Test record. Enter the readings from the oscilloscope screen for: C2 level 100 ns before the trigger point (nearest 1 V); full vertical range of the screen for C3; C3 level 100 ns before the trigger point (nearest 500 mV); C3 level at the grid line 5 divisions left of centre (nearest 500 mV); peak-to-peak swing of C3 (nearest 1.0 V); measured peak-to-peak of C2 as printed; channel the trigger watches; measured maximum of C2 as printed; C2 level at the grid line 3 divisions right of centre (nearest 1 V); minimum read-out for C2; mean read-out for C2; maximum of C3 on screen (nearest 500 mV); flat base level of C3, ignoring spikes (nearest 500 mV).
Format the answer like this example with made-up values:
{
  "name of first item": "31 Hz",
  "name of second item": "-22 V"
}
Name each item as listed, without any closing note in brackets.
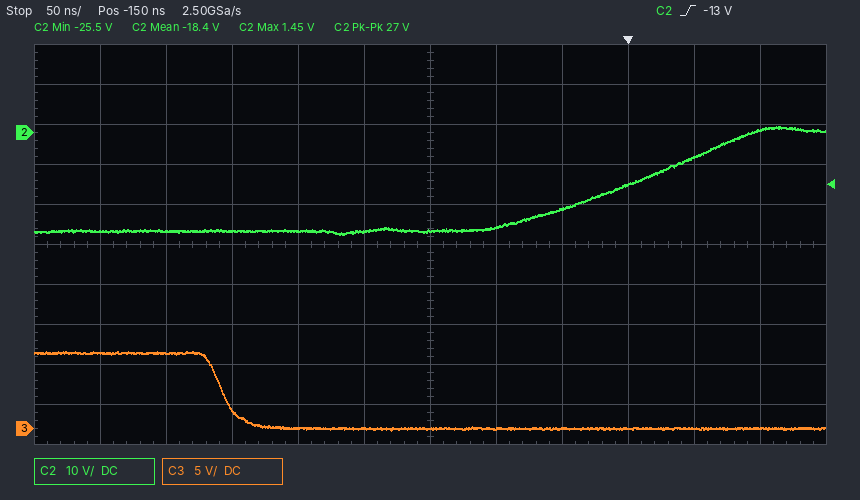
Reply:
{
  "C2 level 100 ns before the trigger point": "-24 V",
  "full vertical range of the screen for C3": "50 V",
  "C3 level 100 ns before the trigger point": "0.0 V",
  "C3 level at the grid line 5 divisions left of centre": "9.5 V",
  "peak-to-peak swing of C3": "10.0 V",
  "measured peak-to-peak of C2 as printed": "27 V",
  "channel the trigger watches": "C2",
  "measured maximum of C2 as printed": "1.45 V",
  "C2 level at the grid line 3 divisions right of centre": "-13 V",
  "minimum read-out for C2": "-25.5 V",
  "mean read-out for C2": "-18.4 V",
  "maximum of C3 on screen": "9.5 V",
  "flat base level of C3, ignoring spikes": "0.0 V"
}
